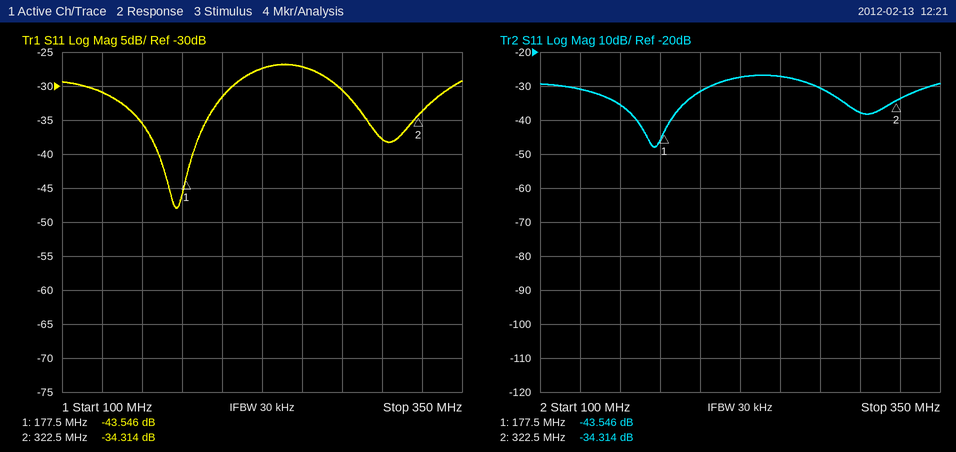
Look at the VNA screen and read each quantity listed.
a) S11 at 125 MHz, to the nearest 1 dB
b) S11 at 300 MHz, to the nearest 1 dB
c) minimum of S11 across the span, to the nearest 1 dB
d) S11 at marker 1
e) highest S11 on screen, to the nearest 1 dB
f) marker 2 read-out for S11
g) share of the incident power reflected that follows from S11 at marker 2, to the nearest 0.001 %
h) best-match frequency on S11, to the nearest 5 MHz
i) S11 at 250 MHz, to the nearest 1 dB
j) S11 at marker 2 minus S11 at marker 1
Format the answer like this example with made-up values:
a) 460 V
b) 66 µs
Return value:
a) -31 dB
b) -38 dB
c) -48 dB
d) -43.546 dB
e) -27 dB
f) -34.314 dB
g) 0.037 %
h) 170 MHz
i) -27 dB
j) 9.232 dB
